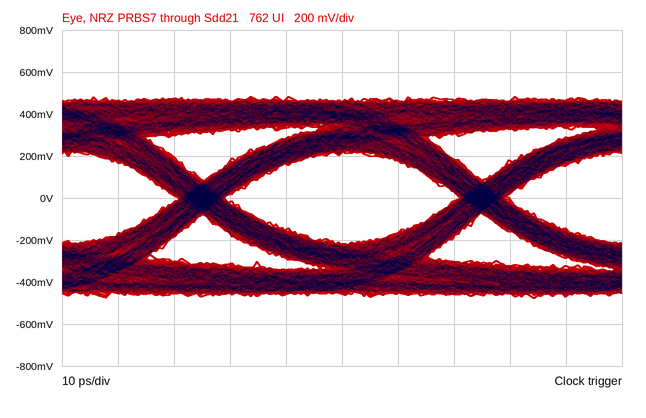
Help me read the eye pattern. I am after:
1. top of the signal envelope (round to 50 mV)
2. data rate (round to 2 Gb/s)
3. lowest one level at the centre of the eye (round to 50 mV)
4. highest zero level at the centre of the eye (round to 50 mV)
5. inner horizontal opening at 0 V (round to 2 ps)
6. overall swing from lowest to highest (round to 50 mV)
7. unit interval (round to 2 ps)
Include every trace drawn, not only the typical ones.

500 mV
20 Gb/s
200 mV
-200 mV
42 ps
950 mV
50 ps
